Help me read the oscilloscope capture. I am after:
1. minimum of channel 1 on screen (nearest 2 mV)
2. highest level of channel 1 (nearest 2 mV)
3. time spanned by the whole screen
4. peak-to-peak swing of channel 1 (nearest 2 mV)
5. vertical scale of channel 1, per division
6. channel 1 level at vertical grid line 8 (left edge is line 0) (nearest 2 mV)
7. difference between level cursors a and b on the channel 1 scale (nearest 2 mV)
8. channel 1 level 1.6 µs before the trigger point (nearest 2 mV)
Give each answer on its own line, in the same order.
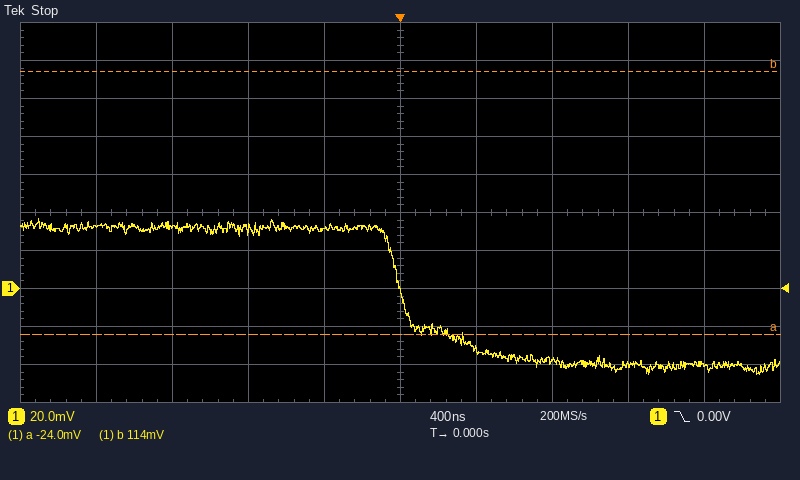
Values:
-46 mV
36 mV
4 µs
82 mV
20 mV
-40 mV
138 mV
32 mV
